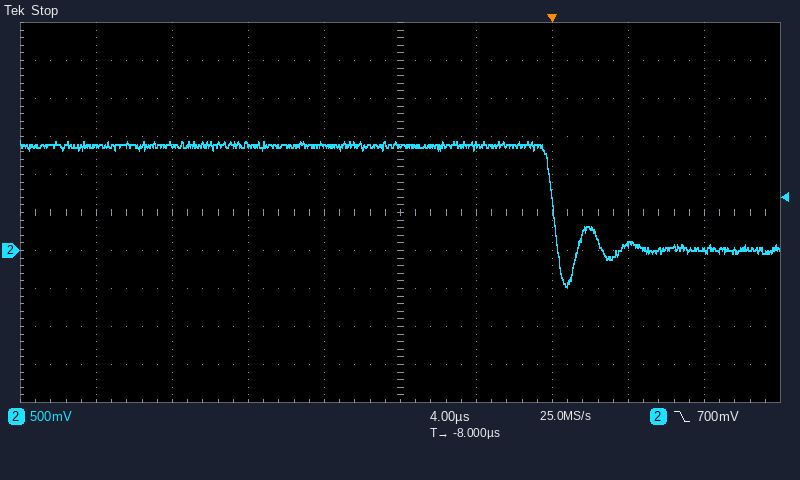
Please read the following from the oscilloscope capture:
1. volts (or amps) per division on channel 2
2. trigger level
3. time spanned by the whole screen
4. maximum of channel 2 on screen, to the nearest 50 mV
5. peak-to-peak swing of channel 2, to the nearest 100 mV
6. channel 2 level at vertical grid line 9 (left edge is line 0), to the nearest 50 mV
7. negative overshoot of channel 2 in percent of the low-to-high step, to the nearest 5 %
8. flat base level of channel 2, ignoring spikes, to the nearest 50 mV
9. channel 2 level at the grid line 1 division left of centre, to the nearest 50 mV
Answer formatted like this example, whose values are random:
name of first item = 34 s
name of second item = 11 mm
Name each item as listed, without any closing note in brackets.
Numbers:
volts (or amps) per division on channel 2 = 500 mV
trigger level = 700 mV
time spanned by the whole screen = 40 µs
maximum of channel 2 on screen, to the nearest 50 mV = 1.45 V
peak-to-peak swing of channel 2, to the nearest 100 mV = 1.90 V
channel 2 level at vertical grid line 9 (left edge is line 0), to the nearest 50 mV = 0 mV
negative overshoot of channel 2 in percent of the low-to-high step, to the nearest 5 % = 35 %
flat base level of channel 2, ignoring spikes, to the nearest 50 mV = 0 mV
channel 2 level at the grid line 1 division left of centre, to the nearest 50 mV = 1.40 V
